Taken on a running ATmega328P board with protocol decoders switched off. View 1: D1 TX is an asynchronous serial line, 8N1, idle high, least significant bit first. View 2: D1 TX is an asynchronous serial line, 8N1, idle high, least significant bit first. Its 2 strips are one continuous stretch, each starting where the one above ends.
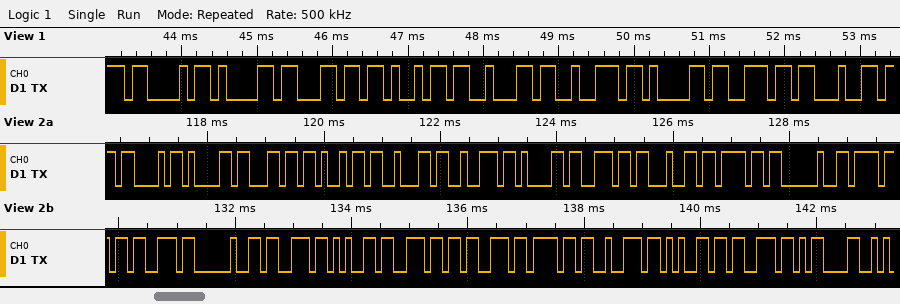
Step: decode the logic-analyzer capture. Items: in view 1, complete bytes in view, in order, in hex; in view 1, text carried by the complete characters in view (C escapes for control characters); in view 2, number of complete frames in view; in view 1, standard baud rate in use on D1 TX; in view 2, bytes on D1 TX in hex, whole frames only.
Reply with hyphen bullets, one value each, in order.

- 0x43 0x61 0x6C 0x69 0x62 0x72 0x61 0x6E 0x64
- "Calibrand"
- 23
- 9600 baud
- 43 61 6C 69 62 72 61 6E 64 6F 20 6F 73 20 73 65 6E 73 6F 72 65 73 0D
